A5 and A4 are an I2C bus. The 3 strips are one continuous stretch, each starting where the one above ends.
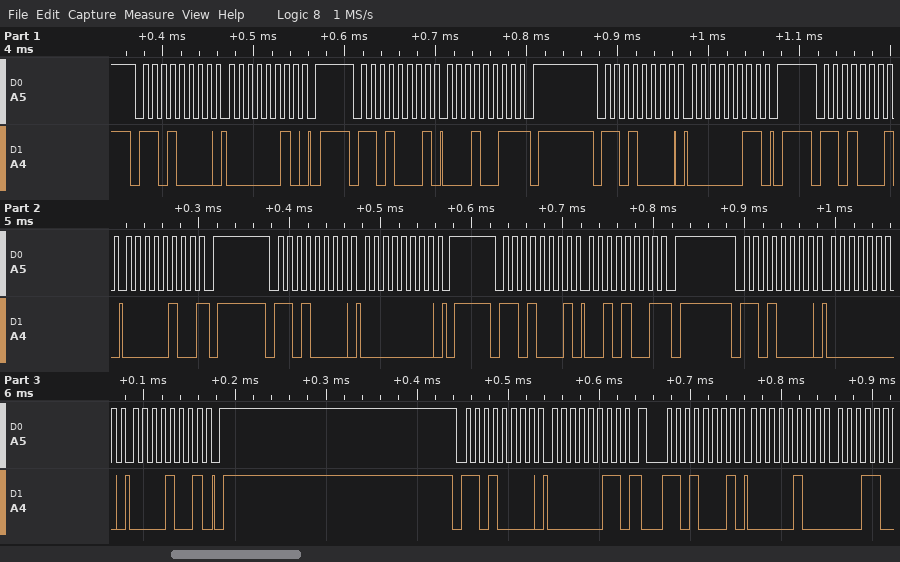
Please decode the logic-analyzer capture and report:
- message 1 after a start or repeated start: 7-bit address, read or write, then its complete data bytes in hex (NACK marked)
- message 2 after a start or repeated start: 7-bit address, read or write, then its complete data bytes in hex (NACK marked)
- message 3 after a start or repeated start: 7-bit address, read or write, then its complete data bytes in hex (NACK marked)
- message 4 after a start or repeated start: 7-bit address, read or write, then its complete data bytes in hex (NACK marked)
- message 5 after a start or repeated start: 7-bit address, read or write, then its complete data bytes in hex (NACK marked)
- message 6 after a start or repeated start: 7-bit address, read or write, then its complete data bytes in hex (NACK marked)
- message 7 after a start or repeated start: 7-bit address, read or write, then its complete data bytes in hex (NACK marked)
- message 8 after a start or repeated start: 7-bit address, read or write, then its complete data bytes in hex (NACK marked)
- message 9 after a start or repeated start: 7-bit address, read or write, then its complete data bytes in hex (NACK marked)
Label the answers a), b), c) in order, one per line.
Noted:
a) 0x68 write: 02
b) 0x68 read: 13 NACK
c) 0x68 write: 03
d) 0x68 read: 04 NACK
e) 0x68 write: 00
f) 0x68 read: 29 NACK
g) 0x68 write: 00 09
h) 0x68 write: 03
i) 0x68 read: 04
